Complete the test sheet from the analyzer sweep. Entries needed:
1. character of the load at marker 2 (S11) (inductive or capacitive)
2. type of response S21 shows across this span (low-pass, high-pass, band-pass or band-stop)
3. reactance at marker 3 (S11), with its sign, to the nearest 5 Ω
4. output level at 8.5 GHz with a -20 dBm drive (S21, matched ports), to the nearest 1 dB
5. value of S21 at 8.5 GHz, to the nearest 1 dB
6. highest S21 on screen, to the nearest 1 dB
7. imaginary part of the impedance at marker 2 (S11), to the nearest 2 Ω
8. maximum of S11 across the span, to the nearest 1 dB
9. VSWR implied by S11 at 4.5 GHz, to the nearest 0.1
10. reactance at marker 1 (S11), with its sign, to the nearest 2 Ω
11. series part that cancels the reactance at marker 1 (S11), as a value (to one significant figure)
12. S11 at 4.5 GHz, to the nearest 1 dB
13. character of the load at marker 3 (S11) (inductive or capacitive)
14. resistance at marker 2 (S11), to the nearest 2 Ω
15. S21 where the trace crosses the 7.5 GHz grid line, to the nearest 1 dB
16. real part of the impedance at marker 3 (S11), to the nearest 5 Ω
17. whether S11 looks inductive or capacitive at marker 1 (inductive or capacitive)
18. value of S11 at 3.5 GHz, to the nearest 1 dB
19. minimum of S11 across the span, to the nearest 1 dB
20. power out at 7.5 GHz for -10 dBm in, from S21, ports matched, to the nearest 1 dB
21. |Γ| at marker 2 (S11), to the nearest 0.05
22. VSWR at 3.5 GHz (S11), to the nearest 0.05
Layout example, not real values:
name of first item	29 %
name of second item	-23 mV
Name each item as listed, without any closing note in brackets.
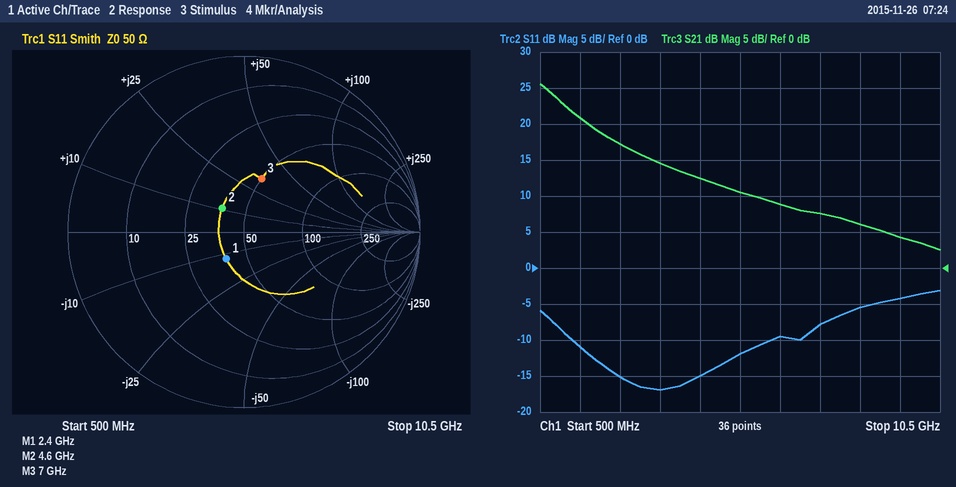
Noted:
character of the load at marker 2 (S11)	inductive
type of response S21 shows across this span	low-pass
reactance at marker 3 (S11), with its sign, to the nearest 5 Ω	+35 Ω
output level at 8.5 GHz with a -20 dBm drive (S21, matched ports), to the nearest 1 dB	-14 dBm
value of S21 at 8.5 GHz, to the nearest 1 dB	6 dB
highest S21 on screen, to the nearest 1 dB	26 dB
imaginary part of the impedance at marker 2 (S11), to the nearest 2 Ω	+10 Ω
maximum of S11 across the span, to the nearest 1 dB	-3 dB
VSWR implied by S11 at 4.5 GHz, to the nearest 0.1	1.4
reactance at marker 1 (S11), with its sign, to the nearest 2 Ω	-12 Ω
series part that cancels the reactance at marker 1 (S11), as a value	800 pH
S11 at 4.5 GHz, to the nearest 1 dB	-15 dB
character of the load at marker 3 (S11)	inductive
resistance at marker 2 (S11), to the nearest 2 Ω	38 Ω
S21 where the trace crosses the 7.5 GHz grid line, to the nearest 1 dB	8 dB
real part of the impedance at marker 3 (S11), to the nearest 5 Ω	50 Ω
whether S11 looks inductive or capacitive at marker 1	capacitive
value of S11 at 3.5 GHz, to the nearest 1 dB	-17 dB
minimum of S11 across the span, to the nearest 1 dB	-17 dB
power out at 7.5 GHz for -10 dBm in, from S21, ports matched, to the nearest 1 dB	-2 dBm
|Γ| at marker 2 (S11), to the nearest 0.05	0.20
VSWR at 3.5 GHz (S11), to the nearest 0.05	1.35
